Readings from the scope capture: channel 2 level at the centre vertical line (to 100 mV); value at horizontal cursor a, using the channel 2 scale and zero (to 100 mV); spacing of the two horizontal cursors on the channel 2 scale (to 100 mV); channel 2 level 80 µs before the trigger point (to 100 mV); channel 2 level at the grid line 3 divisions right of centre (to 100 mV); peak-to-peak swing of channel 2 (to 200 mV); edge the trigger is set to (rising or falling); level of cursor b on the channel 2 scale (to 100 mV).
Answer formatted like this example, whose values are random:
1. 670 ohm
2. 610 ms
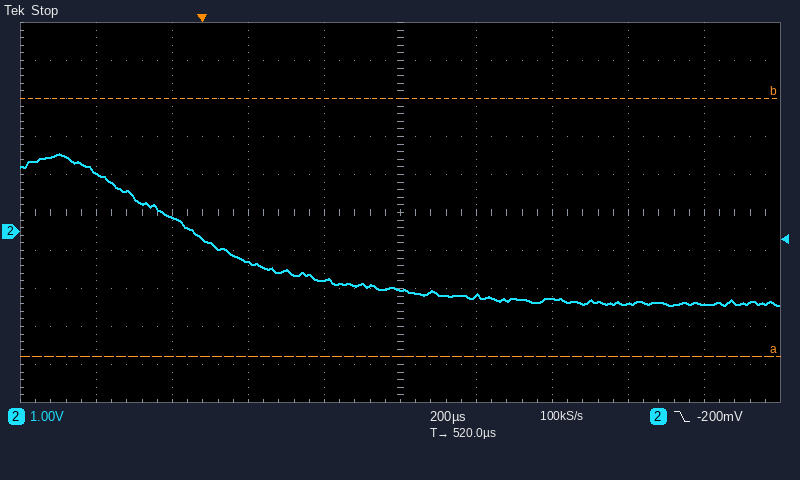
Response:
1. -1.5 V
2. -3.3 V
3. 6.8 V
4. 400 mV
5. -1.9 V
6. 4.0 V
7. falling
8. 3.5 V
